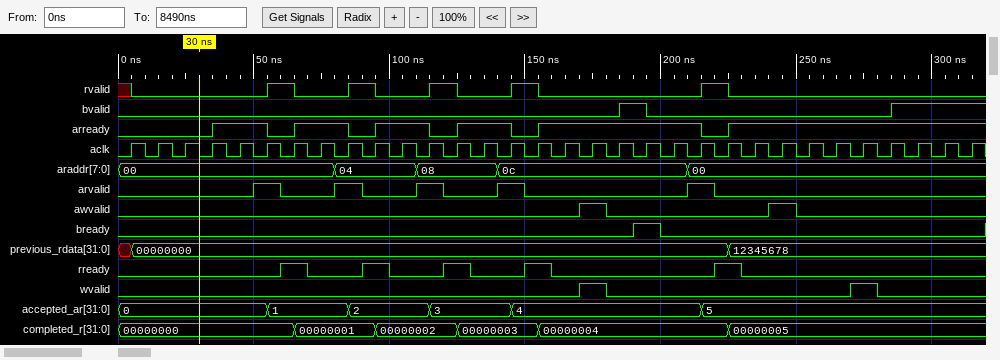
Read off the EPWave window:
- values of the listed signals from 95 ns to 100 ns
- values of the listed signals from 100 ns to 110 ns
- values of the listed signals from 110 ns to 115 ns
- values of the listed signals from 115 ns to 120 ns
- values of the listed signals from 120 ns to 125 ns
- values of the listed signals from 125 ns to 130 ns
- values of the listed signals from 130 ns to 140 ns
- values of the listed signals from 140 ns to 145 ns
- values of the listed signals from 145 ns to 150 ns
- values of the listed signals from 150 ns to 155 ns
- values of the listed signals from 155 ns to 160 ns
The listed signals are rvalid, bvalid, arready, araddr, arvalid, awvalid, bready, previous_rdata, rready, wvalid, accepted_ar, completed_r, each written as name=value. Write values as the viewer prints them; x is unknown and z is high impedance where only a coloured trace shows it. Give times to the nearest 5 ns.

rvalid=0, bvalid=0, arready=1, araddr=04, arvalid=0, awvalid=0, bready=0, previous_rdata=00000000, rready=1, wvalid=0, accepted_ar=2, completed_r=00000002
rvalid=0, bvalid=0, arready=1, araddr=04, arvalid=0, awvalid=0, bready=0, previous_rdata=00000000, rready=0, wvalid=0, accepted_ar=2, completed_r=00000002
rvalid=0, bvalid=0, arready=1, araddr=08, arvalid=1, awvalid=0, bready=0, previous_rdata=00000000, rready=0, wvalid=0, accepted_ar=2, completed_r=00000002
rvalid=1, bvalid=0, arready=0, araddr=08, arvalid=1, awvalid=0, bready=0, previous_rdata=00000000, rready=0, wvalid=0, accepted_ar=3, completed_r=00000002
rvalid=1, bvalid=0, arready=0, araddr=08, arvalid=0, awvalid=0, bready=0, previous_rdata=00000000, rready=1, wvalid=0, accepted_ar=3, completed_r=00000002
rvalid=0, bvalid=0, arready=1, araddr=08, arvalid=0, awvalid=0, bready=0, previous_rdata=00000000, rready=1, wvalid=0, accepted_ar=3, completed_r=00000003
rvalid=0, bvalid=0, arready=1, araddr=08, arvalid=0, awvalid=0, bready=0, previous_rdata=00000000, rready=0, wvalid=0, accepted_ar=3, completed_r=00000003
rvalid=0, bvalid=0, arready=1, araddr=0c, arvalid=1, awvalid=0, bready=0, previous_rdata=00000000, rready=0, wvalid=0, accepted_ar=3, completed_r=00000003
rvalid=1, bvalid=0, arready=0, araddr=0c, arvalid=1, awvalid=0, bready=0, previous_rdata=00000000, rready=0, wvalid=0, accepted_ar=4, completed_r=00000003
rvalid=1, bvalid=0, arready=0, araddr=0c, arvalid=0, awvalid=0, bready=0, previous_rdata=00000000, rready=1, wvalid=0, accepted_ar=4, completed_r=00000003
rvalid=0, bvalid=0, arready=1, araddr=0c, arvalid=0, awvalid=0, bready=0, previous_rdata=00000000, rready=1, wvalid=0, accepted_ar=4, completed_r=00000004
